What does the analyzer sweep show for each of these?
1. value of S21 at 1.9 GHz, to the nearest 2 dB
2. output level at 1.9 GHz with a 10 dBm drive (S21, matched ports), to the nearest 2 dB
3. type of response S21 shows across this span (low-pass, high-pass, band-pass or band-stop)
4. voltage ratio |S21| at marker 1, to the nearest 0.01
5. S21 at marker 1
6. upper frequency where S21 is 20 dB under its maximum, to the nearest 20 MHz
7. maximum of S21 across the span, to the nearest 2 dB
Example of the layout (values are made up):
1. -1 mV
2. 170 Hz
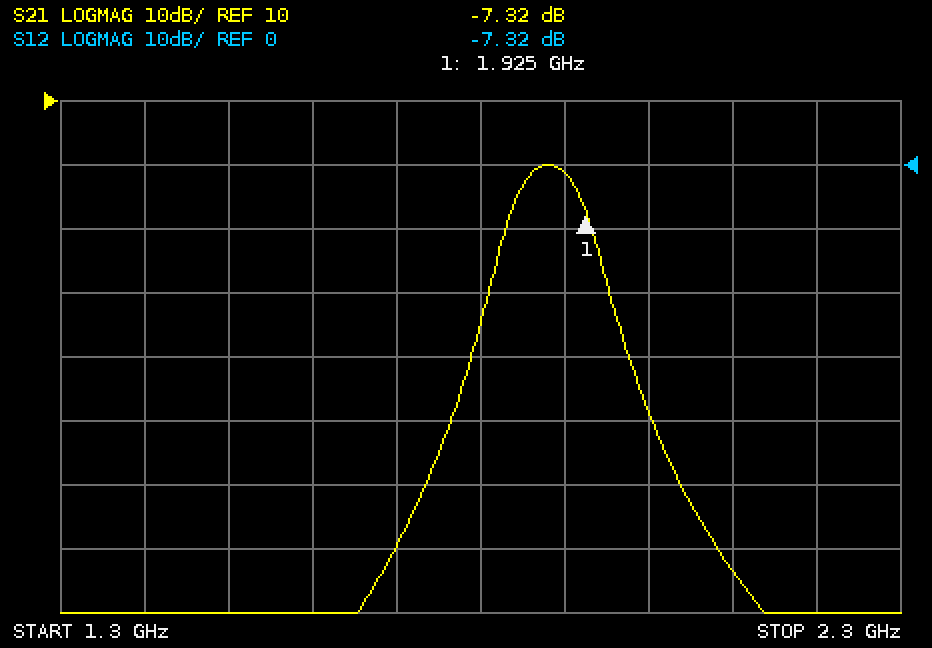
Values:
1. -2 dB
2. 8 dBm
3. band-pass
4. 0.43
5. -7.32 dB
6. 1.96 GHz
7. 0 dB
